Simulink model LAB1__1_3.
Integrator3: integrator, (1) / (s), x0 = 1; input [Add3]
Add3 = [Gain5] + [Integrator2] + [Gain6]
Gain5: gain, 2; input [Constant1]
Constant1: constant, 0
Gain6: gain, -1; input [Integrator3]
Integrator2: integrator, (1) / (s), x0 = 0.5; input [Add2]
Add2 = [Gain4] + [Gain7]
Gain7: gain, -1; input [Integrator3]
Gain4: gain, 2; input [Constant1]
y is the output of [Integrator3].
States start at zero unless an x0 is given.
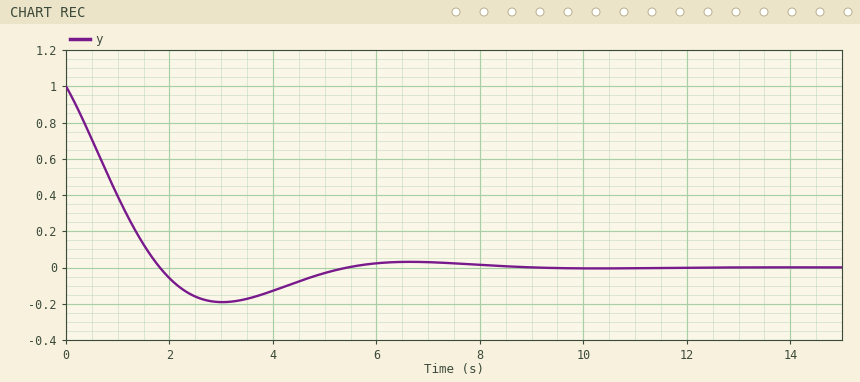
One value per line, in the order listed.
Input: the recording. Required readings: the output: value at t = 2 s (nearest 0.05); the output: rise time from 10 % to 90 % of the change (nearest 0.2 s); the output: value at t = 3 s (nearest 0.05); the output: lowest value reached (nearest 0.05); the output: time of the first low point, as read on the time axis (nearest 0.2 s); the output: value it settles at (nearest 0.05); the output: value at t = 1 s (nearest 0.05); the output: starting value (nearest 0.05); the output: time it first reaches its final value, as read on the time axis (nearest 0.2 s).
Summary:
-0.05
1.4 s
-0.20
-0.20
3.0 s
0.00
0.40
1.00
1.8 s
